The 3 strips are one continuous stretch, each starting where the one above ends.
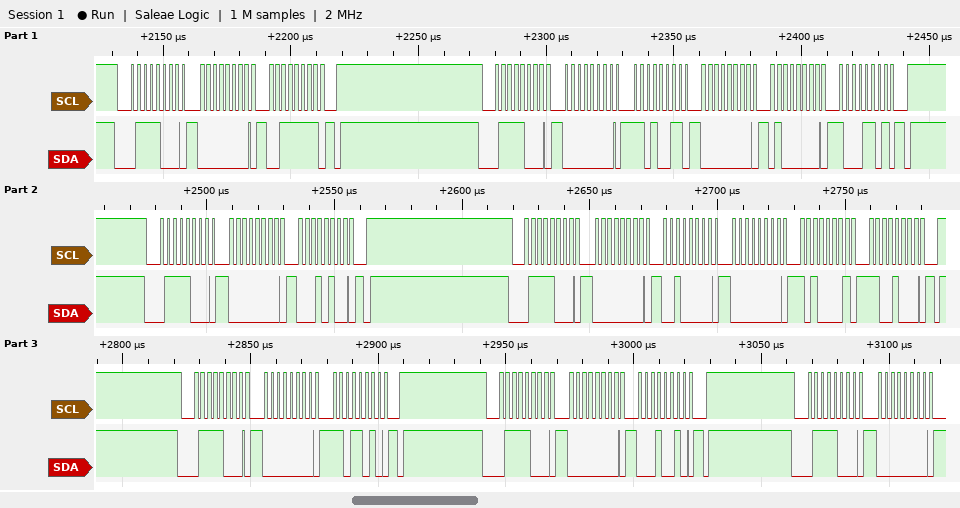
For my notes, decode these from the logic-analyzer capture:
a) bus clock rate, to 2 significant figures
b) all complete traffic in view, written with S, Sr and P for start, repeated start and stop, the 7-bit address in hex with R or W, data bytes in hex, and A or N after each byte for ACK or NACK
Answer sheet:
400 kHz
S 3CW A 00 A 3F A P S 3CW A 00 A D3 A 00 A 40 A 8D A P S 3CW A 00 A 14 A P S 3CW A 00 A 20 A 00 A A1 A C8 A P S 3CW A 00 A DA A P S 3CW A 00 A 12 A P S 3CW A 00 A
